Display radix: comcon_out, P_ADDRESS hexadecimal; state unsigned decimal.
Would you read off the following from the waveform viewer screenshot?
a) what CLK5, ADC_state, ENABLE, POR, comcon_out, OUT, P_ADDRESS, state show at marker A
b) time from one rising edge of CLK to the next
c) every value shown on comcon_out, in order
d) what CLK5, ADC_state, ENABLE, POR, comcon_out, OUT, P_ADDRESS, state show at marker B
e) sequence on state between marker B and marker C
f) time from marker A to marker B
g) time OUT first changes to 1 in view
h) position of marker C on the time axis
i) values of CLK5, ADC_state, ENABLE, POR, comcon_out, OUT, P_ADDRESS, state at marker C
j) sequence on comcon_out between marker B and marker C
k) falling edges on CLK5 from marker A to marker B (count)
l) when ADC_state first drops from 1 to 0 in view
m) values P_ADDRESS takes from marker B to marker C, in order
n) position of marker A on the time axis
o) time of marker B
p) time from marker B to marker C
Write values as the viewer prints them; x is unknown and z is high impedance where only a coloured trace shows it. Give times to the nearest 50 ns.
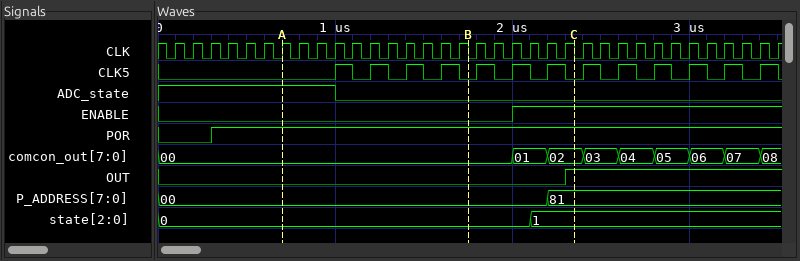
CLK5=0, ADC_state=1, ENABLE=0, POR=1, comcon_out=00, OUT=0, P_ADDRESS=00, state=0
100 ns
00, 01, 02, 03, 04, 05, 06, 07, 08
CLK5=0, ADC_state=0, ENABLE=0, POR=1, comcon_out=00, OUT=0, P_ADDRESS=00, state=0
0, 1
1050 ns
2300 ns
2350 ns
CLK5=0, ADC_state=0, ENABLE=1, POR=1, comcon_out=02, OUT=1, P_ADDRESS=81, state=1
00, 01, 02
4
1000 ns
00, 81
700 ns
1750 ns
600 ns
